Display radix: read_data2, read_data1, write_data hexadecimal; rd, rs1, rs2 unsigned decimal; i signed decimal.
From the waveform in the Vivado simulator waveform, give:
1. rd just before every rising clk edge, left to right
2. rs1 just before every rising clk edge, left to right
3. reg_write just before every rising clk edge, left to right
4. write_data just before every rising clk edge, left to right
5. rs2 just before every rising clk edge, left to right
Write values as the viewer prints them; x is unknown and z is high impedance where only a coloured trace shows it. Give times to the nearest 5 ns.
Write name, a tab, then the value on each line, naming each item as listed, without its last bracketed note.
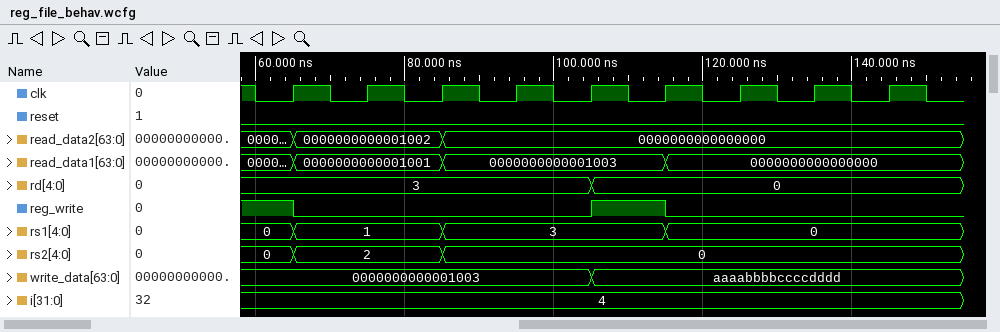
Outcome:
rd just before every rising clk edge, left to right	3, 3, 3, 3, 3, 0, 0, 0, 0
rs1 just before every rising clk edge, left to right	0, 1, 1, 3, 3, 3, 0, 0, 0
reg_write just before every rising clk edge, left to right	1 0 0 0 0 1 0 0 0
write_data just before every rising clk edge, left to right	0000000000001003, 0000000000001003, 0000000000001003, 0000000000001003, 0000000000001003, aaaabbbbccccdddd, aaaabbbbccccdddd, aaaabbbbccccdddd, aaaabbbbccccdddd
rs2 just before every rising clk edge, left to right	0, 2, 2, 0, 0, 0, 0, 0, 0
